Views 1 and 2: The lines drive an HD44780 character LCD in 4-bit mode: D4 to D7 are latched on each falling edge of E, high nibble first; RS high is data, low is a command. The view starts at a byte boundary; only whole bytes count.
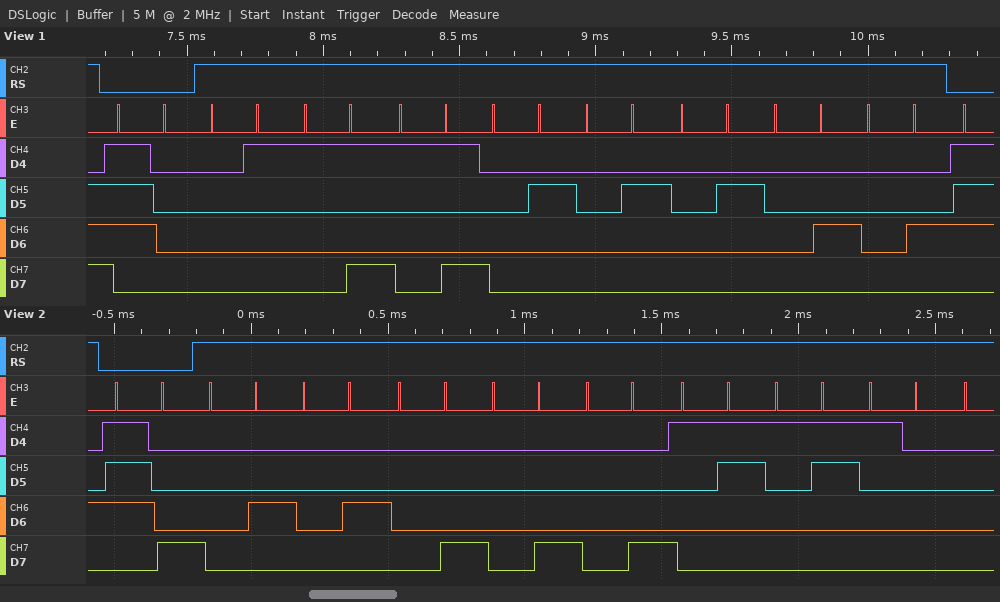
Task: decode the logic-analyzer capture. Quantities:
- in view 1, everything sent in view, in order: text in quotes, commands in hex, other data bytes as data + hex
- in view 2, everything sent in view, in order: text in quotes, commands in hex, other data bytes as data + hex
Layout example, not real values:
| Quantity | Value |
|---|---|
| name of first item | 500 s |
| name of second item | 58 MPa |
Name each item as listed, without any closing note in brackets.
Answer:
| Quantity | Value |
|---|---|
| in view 1, everything sent in view, in order: text in quotes, commands in hex, other data bytes as data + hex | 0x70 data 01 19 19 02 02 02 04 04 |
| in view 2, everything sent in view, in order: text in quotes, commands in hex, other data bytes as data + hex | 0x78 data 04 04 08 08 08 13 13 10 |
